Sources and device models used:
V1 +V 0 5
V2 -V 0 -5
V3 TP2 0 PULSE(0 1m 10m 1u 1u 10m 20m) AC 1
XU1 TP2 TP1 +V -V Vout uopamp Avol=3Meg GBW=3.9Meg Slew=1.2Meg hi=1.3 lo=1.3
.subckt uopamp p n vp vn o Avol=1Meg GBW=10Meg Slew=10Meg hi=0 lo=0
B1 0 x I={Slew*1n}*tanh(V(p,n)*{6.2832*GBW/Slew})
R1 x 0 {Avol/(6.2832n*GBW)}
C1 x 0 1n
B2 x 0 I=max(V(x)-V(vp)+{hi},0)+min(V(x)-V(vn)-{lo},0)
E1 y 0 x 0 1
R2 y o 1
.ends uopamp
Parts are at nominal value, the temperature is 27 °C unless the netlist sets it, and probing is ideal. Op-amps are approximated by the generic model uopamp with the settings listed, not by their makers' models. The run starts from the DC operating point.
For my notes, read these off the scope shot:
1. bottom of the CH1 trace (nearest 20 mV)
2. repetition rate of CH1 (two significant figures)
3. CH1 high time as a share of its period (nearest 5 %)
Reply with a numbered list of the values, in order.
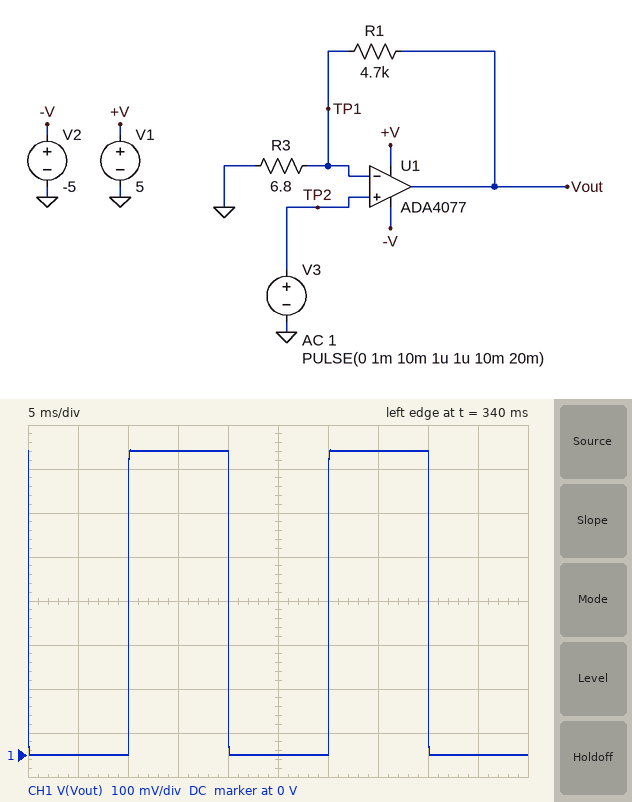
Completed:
1. 0 V
2. 50 Hz
3. 50 %
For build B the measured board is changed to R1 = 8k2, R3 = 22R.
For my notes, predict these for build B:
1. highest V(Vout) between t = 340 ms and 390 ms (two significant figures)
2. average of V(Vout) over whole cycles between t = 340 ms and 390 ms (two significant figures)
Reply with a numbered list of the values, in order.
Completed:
1. 370 mV
2. 190 mV
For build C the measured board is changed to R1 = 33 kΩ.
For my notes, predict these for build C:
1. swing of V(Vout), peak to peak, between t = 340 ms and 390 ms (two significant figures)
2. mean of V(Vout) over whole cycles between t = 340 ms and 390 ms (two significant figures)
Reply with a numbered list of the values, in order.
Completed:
1. 3.7 V
2. 1.9 V
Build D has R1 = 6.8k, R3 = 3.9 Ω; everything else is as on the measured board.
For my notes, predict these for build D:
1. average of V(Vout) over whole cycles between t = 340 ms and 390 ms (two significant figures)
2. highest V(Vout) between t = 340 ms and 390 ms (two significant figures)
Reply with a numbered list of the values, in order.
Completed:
1. 870 mV
2. 1.7 V
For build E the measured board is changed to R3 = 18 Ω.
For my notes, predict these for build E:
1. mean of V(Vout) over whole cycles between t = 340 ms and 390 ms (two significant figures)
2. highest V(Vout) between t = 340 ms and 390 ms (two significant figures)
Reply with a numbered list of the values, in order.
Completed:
1. 130 mV
2. 260 mV
